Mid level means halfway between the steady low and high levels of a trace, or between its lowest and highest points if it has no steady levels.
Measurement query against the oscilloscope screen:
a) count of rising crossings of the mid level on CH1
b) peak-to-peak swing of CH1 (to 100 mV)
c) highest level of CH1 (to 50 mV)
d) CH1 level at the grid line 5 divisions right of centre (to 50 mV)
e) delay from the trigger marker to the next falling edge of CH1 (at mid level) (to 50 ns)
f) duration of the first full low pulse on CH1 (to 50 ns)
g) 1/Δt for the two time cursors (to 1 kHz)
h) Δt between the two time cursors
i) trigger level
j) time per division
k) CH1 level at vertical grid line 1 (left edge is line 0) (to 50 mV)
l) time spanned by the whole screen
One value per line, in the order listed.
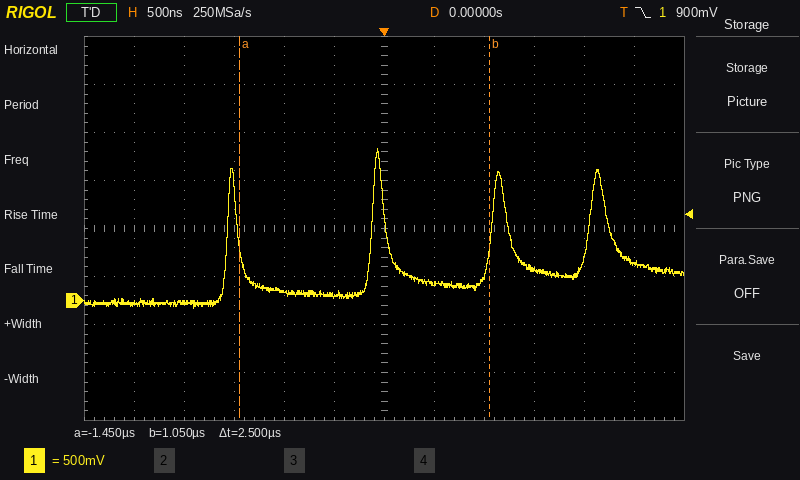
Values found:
4
1.70 V
1.60 V
400 mV
1.25 µs
1.35 µs
400 kHz
2.5 µs
900 mV
500 ns
-50 mV
6 µs
